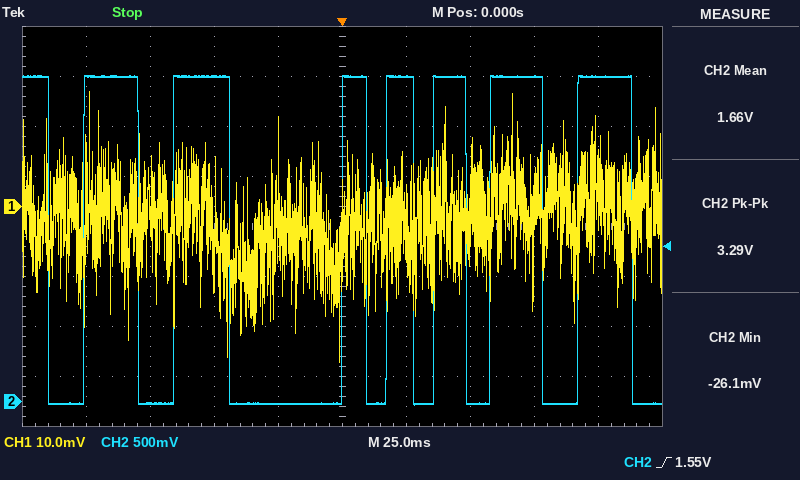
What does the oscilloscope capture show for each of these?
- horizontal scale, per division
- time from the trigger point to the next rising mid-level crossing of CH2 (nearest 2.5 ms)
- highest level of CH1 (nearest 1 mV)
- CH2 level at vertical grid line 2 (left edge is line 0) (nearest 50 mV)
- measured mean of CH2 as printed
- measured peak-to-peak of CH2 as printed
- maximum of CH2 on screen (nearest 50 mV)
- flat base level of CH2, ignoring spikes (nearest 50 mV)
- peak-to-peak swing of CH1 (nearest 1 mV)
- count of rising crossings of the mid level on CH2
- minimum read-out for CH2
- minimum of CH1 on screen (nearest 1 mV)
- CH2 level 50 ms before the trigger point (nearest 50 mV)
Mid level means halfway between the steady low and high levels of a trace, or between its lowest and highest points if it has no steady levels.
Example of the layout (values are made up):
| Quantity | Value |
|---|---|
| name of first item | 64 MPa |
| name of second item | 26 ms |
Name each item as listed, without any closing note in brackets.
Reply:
| Quantity | Value |
|---|---|
| horizontal scale, per division | 25 ms |
| time from the trigger point to the next rising mid-level crossing of CH2 | 17.5 ms |
| highest level of CH1 | 23 mV |
| CH2 level at vertical grid line 2 (left edge is line 0) | 0 mV |
| measured mean of CH2 as printed | 1.66 V |
| measured peak-to-peak of CH2 as printed | 3.29 V |
| maximum of CH2 on screen | 3.25 V |
| flat base level of CH2, ignoring spikes | 0 mV |
| peak-to-peak swing of CH1 | 54 mV |
| count of rising crossings of the mid level on CH2 | 7 |
| minimum read-out for CH2 | -26.1 mV |
| minimum of CH1 on screen | -31 mV |
| CH2 level 50 ms before the trigger point | 3.25 V |
